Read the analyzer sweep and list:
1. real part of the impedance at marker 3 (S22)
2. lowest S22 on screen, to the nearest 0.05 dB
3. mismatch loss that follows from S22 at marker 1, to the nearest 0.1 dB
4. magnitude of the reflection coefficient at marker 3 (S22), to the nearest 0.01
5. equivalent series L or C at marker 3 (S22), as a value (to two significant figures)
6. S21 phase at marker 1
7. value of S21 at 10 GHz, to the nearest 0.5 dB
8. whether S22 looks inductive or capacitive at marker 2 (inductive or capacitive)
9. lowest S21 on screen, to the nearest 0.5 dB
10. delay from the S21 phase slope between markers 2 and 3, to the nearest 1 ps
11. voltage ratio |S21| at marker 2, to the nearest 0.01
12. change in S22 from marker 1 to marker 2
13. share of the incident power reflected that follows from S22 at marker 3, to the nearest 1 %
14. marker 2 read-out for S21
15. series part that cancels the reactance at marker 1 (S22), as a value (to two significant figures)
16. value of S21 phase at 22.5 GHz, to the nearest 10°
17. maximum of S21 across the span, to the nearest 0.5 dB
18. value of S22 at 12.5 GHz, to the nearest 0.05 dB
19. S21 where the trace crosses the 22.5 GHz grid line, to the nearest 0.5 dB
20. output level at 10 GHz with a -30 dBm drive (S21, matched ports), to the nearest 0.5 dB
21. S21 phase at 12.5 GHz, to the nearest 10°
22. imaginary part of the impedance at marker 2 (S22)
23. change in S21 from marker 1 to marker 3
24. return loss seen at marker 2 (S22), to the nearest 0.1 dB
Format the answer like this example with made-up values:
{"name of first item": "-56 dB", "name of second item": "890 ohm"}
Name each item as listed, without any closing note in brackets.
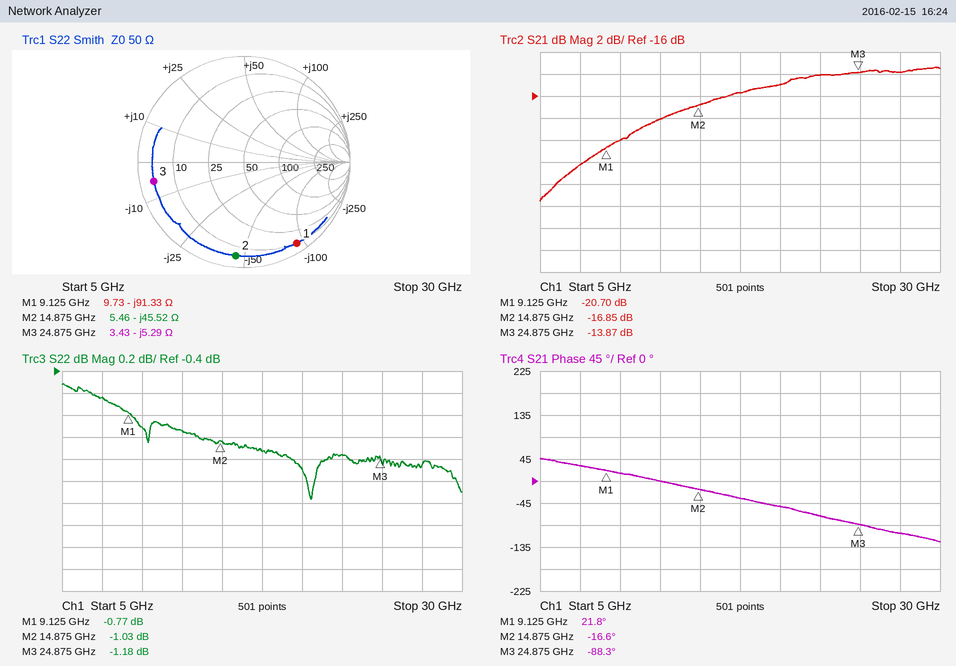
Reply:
{"real part of the impedance at marker 3": "3.43 Ω", "lowest S22 on screen, to the nearest 0.05 dB": "-1.55 dB", "mismatch loss that follows from S22 at marker 1, to the nearest 0.1 dB": "7.9 dB", "magnitude of the reflection coefficient at marker 3 (S22), to the nearest 0.01": "0.87", "equivalent series L or C at marker 3 (S22), as a value": "1.2 pF", "S21 phase at marker 1": "21.8°", "value of S21 at 10 GHz, to the nearest 0.5 dB": "-20.0 dB", "whether S22 looks inductive or capacitive at marker 2": "capacitive", "lowest S21 on screen, to the nearest 0.5 dB": "-25.5 dB", "delay from the S21 phase slope between markers 2 and 3, to the nearest 1 ps": "20 ps", "voltage ratio |S21| at marker 2, to the nearest 0.01": "0.14", "change in S22 from marker 1 to marker 2": "-0.26 dB", "share of the incident power reflected that follows from S22 at marker 3, to the nearest 1 %": "76 %", "marker 2 read-out for S21": "-16.85 dB", "series part that cancels the reactance at marker 1 (S22), as a value": "1.6 nH", "value of S21 phase at 22.5 GHz, to the nearest 10°": "-70°", "maximum of S21 across the span, to the nearest 0.5 dB": "-13.5 dB", "value of S22 at 12.5 GHz, to the nearest 0.05 dB": "-0.95 dB", "S21 where the trace crosses the 22.5 GHz grid line, to the nearest 0.5 dB": "-14.0 dB", "output level at 10 GHz with a -30 dBm drive (S21, matched ports), to the nearest 0.5 dB": "-50.0 dBm", "S21 phase at 12.5 GHz, to the nearest 10°": "0°", "imaginary part of the impedance at marker 2": "-45.52 Ω", "change in S21 from marker 1 to marker 3": "6.83 dB", "return loss seen at marker 2 (S22), to the nearest 0.1 dB": "1.0 dB"}
